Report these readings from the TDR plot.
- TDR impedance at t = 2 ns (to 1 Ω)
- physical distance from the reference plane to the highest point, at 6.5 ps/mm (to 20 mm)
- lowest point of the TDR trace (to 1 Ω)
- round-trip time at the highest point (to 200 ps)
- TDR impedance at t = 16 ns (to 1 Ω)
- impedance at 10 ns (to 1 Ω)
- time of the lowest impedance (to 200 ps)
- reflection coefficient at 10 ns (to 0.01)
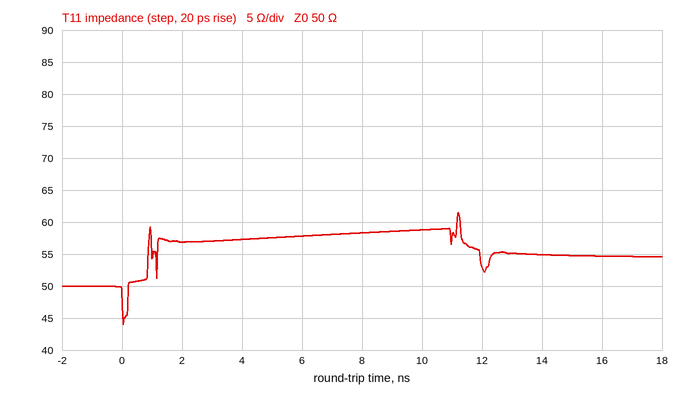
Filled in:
57 Ω
860 mm
44 Ω
11.2 ns
55 Ω
59 Ω
0.0 ns
+0.08
